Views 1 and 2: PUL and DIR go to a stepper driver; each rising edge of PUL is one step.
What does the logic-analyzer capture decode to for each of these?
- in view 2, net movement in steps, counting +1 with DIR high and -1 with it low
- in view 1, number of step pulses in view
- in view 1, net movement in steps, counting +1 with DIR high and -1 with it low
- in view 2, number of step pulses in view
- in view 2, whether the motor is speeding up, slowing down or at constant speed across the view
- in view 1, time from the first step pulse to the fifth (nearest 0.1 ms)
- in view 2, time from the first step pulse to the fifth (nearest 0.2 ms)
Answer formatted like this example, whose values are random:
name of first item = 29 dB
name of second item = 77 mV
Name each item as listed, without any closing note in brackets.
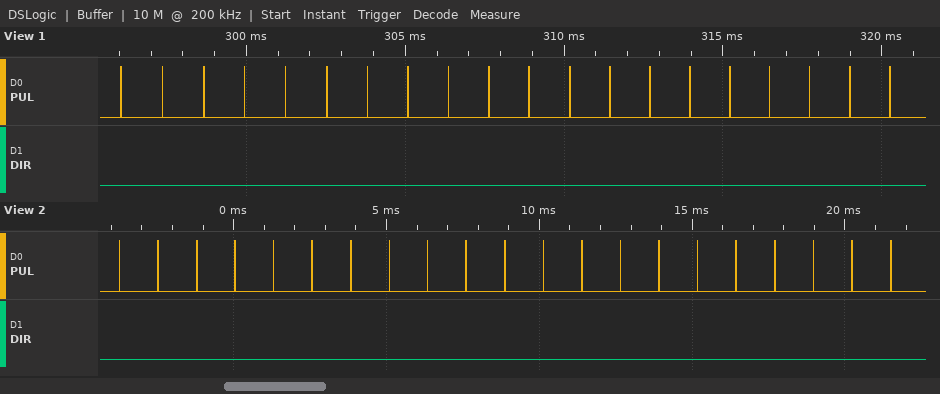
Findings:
in view 2, net movement in steps, counting +1 with DIR high and -1 with it low = -21
in view 1, number of step pulses in view = 20
in view 1, net movement in steps, counting +1 with DIR high and -1 with it low = -20
in view 2, number of step pulses in view = 21
in view 2, whether the motor is speeding up, slowing down or at constant speed across the view = constant speed
in view 1, time from the first step pulse to the fifth = 5.2 ms
in view 2, time from the first step pulse to the fifth = 5.0 ms
